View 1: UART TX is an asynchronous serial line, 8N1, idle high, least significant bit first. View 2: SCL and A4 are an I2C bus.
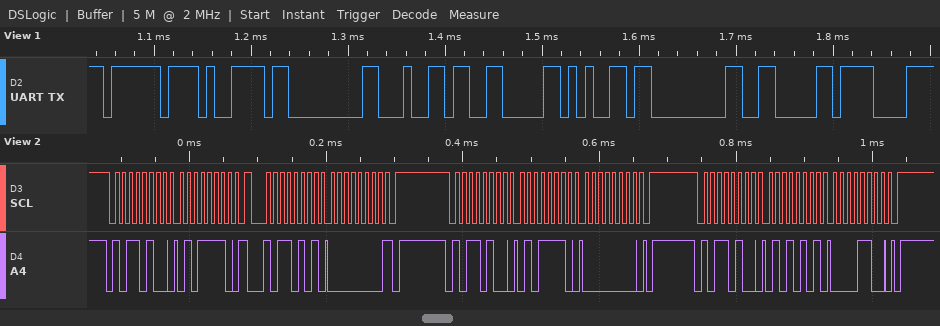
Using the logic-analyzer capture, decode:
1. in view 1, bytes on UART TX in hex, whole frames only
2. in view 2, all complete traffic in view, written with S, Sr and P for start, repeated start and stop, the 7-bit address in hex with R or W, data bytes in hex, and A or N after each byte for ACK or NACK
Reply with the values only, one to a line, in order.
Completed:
BF 79 00 64 06 65 00 06 0F
S 5AW A 5E A Sr 5AR A 00 N P S 5AW A 5E A 00 A P S 5AW A 55 A 0C A P
